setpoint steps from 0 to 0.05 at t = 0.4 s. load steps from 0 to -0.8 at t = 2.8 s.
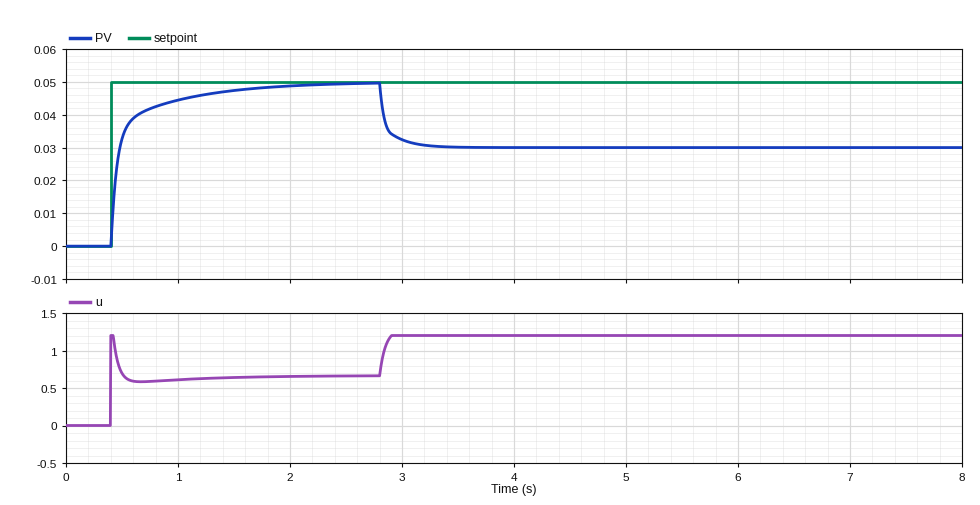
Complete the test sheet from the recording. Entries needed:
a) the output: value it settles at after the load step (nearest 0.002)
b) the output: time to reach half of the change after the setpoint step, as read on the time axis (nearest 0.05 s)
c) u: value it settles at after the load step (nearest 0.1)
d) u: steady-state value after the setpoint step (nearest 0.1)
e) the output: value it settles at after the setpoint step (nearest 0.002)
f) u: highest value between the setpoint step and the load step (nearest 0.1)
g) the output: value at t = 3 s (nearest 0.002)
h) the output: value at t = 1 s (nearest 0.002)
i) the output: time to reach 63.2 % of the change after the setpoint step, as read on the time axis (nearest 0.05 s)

0.030
0.45 s
1.2
0.7
0.050
1.2
0.032
0.044
0.50 s
